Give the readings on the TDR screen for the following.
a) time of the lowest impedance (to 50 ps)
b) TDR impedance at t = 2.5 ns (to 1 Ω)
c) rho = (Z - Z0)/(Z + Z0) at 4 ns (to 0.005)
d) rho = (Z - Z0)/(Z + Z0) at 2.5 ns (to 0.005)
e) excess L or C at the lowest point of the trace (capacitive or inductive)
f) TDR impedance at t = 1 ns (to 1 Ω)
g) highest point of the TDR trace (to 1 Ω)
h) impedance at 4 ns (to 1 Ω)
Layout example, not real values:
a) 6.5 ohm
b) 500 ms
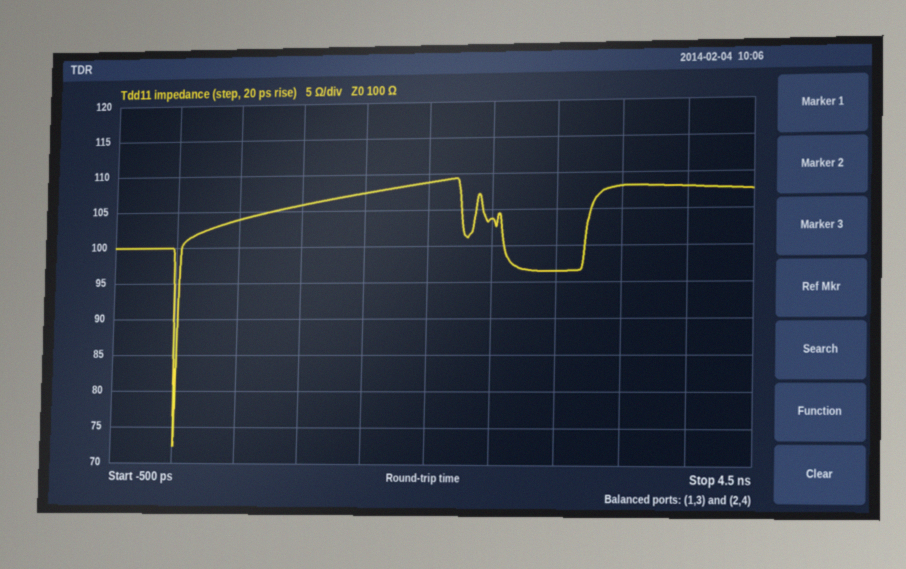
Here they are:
a) 0 ps
b) 104 Ω
c) +0.040
d) +0.020
e) capacitive
f) 106 Ω
g) 109 Ω
h) 108 Ω
